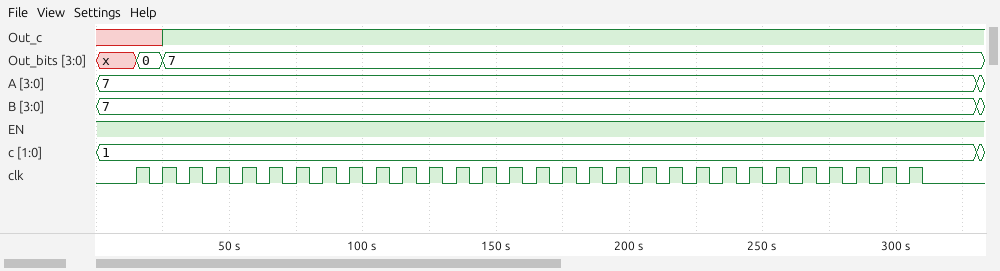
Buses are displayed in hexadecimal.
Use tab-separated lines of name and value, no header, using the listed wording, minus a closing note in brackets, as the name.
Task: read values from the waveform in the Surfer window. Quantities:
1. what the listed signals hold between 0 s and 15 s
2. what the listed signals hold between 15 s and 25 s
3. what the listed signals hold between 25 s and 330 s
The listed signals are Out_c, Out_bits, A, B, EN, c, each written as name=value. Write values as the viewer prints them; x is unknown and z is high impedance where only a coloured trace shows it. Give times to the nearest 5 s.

what the listed signals hold between 0 s and 15 s	Out_c=x, Out_bits=x, A=7, B=7, EN=1, c=1
what the listed signals hold between 15 s and 25 s	Out_c=x, Out_bits=0, A=7, B=7, EN=1, c=1
what the listed signals hold between 25 s and 330 s	Out_c=1, Out_bits=7, A=7, B=7, EN=1, c=1
